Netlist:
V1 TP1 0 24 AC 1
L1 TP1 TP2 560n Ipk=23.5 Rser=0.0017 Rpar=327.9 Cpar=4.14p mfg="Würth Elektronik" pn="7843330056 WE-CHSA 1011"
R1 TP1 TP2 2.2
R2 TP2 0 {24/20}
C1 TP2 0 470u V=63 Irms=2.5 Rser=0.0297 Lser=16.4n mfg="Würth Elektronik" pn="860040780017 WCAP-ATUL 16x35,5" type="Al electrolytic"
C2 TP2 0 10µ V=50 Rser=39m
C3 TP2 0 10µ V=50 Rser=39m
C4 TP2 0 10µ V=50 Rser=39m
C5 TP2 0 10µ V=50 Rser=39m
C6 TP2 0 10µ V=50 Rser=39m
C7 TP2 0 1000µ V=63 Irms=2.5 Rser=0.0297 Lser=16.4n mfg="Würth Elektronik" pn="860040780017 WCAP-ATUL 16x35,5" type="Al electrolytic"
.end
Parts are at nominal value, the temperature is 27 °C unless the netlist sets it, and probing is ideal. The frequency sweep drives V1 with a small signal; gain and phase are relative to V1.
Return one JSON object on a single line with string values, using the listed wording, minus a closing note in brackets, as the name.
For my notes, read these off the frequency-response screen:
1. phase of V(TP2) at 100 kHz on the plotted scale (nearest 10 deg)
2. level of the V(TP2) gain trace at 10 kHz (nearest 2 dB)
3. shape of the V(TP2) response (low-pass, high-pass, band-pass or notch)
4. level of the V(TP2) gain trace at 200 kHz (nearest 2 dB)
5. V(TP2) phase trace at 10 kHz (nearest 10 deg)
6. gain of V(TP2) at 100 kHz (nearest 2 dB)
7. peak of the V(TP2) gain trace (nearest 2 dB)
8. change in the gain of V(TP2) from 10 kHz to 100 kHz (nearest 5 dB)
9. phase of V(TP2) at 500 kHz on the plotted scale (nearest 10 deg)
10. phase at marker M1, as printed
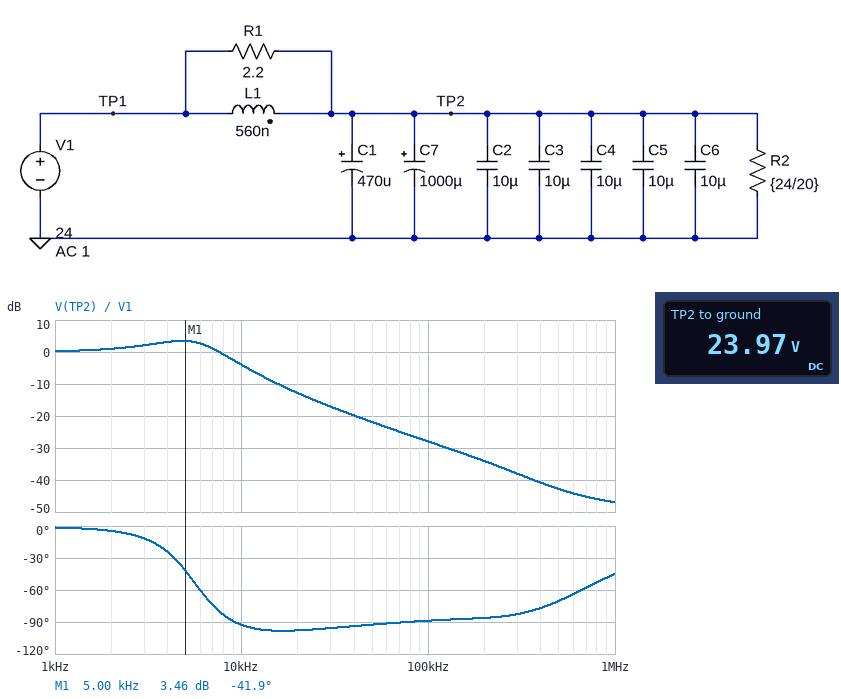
{"phase of V(TP2) at 100 kHz on the plotted scale": "-90 deg", "level of the V(TP2) gain trace at 10 kHz": "-4 dB", "shape of the V(TP2) response": "low-pass", "level of the V(TP2) gain trace at 200 kHz": "-34 dB", "V(TP2) phase trace at 10 kHz": "-90 deg", "gain of V(TP2) at 100 kHz": "-28 dB", "peak of the V(TP2) gain trace": "4 dB", "change in the gain of V(TP2) from 10 kHz to 100 kHz": "-25 dB", "phase of V(TP2) at 500 kHz on the plotted scale": "-70 deg", "phase at marker M1, as printed": "-41.9 deg"}
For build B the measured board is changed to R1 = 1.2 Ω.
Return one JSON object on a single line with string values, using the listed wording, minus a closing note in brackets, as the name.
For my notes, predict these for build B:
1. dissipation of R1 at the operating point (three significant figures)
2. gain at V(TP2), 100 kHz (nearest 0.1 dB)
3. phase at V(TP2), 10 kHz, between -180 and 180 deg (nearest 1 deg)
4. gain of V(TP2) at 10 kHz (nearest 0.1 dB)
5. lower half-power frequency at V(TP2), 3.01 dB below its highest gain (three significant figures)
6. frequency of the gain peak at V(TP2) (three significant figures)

{"dissipation of R1 at the operating point": "958 µW", "gain at V(TP2), 100 kHz": "-27.8 dB", "phase at V(TP2), 10 kHz, between -180 and 180 deg": "-92 deg", "gain of V(TP2) at 10 kHz": "-4.1 dB", "lower half-power frequency at V(TP2), 3.01 dB below its highest gain": "1.29 kHz", "frequency of the gain peak at V(TP2)": "4.79 kHz"}
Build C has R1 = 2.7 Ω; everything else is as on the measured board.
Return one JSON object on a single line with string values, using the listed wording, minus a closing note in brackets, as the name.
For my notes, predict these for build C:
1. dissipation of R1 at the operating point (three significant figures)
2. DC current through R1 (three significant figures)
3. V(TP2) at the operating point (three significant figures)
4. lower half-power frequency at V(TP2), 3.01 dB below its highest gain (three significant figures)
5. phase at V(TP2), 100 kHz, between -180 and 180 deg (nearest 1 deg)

{"dissipation of R1 at the operating point": "426 µW", "DC current through R1": "12.6 mA", "V(TP2) at the operating point": "24.0 V", "lower half-power frequency at V(TP2), 3.01 dB below its highest gain": "1.38 kHz", "phase at V(TP2), 100 kHz, between -180 and 180 deg": "-90 deg"}
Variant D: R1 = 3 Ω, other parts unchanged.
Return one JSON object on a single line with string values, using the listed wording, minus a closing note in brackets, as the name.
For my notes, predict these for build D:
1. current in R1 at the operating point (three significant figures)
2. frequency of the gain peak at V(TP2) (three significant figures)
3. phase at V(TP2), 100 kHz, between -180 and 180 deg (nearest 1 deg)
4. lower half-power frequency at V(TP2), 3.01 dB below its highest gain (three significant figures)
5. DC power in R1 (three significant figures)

{"current in R1 at the operating point": "11.3 mA", "frequency of the gain peak at V(TP2)": "4.82 kHz", "phase at V(TP2), 100 kHz, between -180 and 180 deg": "-91 deg", "lower half-power frequency at V(TP2), 3.01 dB below its highest gain": "1.39 kHz", "DC power in R1": "384 µW"}
